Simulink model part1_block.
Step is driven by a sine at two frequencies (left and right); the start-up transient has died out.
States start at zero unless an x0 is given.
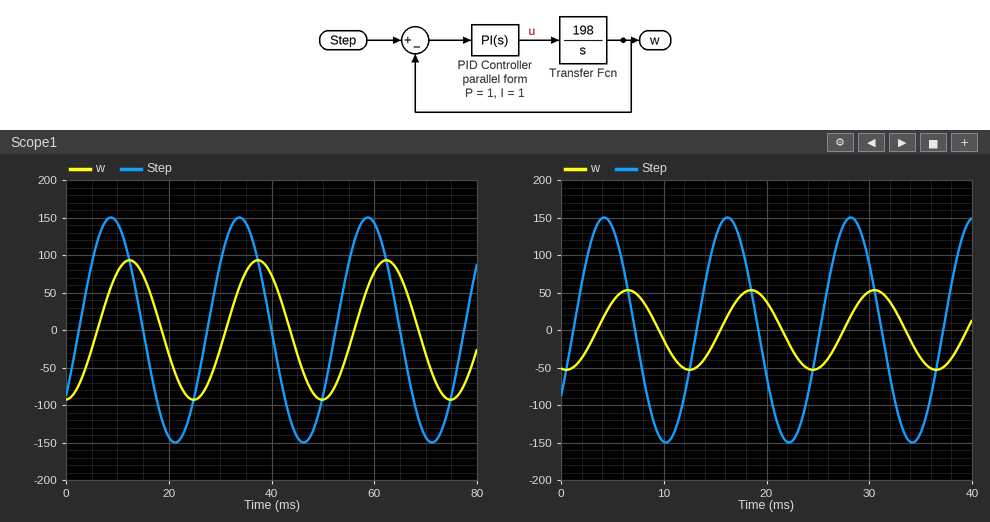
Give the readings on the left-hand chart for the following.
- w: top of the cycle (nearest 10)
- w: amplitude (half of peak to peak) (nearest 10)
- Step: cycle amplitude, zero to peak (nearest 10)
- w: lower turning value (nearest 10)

90
90
150
-90
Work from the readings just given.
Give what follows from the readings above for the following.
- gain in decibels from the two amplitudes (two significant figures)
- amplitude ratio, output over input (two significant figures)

-4.4 dB
0.60
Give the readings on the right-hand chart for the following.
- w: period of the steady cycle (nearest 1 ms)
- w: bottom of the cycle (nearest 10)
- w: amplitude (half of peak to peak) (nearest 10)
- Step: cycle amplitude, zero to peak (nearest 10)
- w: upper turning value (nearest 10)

12 ms
-50
50
150
50
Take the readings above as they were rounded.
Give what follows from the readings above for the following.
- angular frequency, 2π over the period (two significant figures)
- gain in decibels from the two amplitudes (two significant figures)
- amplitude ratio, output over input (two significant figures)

0.52 rad/ms
-9.5 dB
0.33
